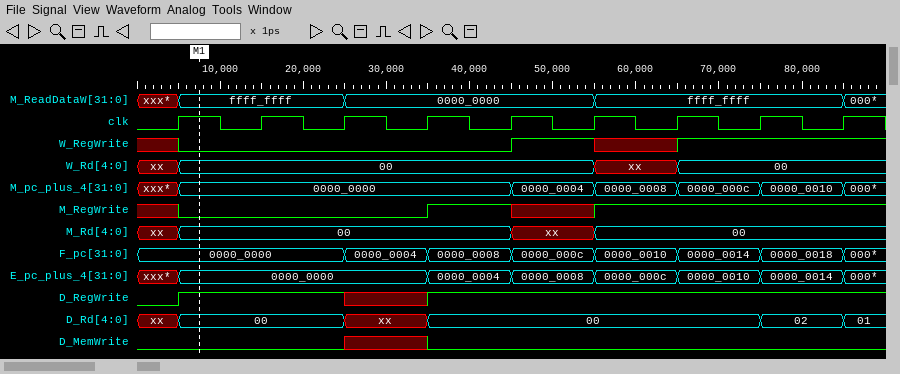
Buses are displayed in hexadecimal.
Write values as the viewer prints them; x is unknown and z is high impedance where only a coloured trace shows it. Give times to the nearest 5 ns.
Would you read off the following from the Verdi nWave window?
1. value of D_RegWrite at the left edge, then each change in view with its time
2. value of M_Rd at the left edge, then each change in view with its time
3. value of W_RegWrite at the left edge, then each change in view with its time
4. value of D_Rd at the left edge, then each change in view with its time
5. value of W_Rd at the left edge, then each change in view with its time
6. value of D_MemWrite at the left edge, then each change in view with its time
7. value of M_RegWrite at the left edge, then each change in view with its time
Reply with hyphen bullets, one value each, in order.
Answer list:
- 0, 1 at 5 ns, x at 25 ns, 1 at 35 ns
- xx, 00 at 5 ns, xx at 45 ns, 00 at 55 ns
- x, 0 at 5 ns, 1 at 45 ns, x at 55 ns, 1 at 65 ns
- xx, 00 at 5 ns, xx at 25 ns, 00 at 35 ns, 02 at 75 ns, 01 at 85 ns
- xx, 00 at 5 ns, xx at 55 ns, 00 at 65 ns
- 0, x at 25 ns, 0 at 35 ns
- x, 0 at 5 ns, 1 at 35 ns, x at 45 ns, 1 at 55 ns
